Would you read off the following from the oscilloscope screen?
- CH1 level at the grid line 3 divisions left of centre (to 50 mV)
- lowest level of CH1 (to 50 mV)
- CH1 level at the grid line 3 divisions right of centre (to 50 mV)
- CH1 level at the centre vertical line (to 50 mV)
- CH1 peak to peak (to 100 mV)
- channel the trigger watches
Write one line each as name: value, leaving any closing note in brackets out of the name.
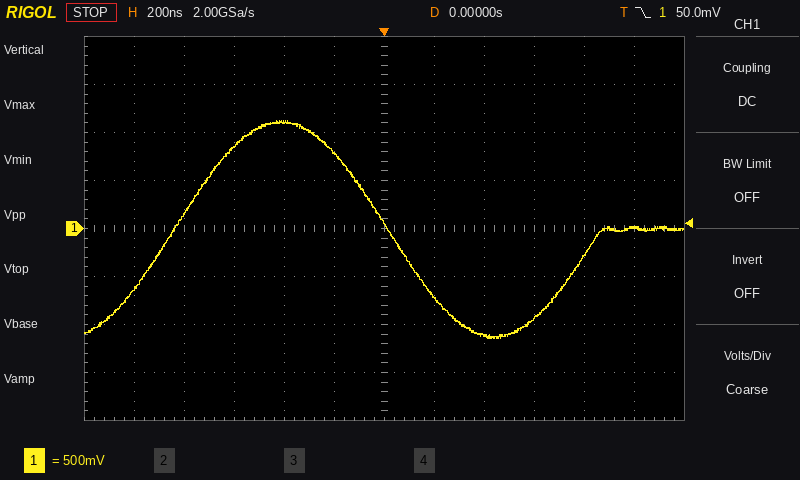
CH1 level at the grid line 3 divisions left of centre: 850 mV
lowest level of CH1: -1.15 V
CH1 level at the grid line 3 divisions right of centre: -950 mV
CH1 level at the centre vertical line: 50 mV
CH1 peak to peak: 2.30 V
channel the trigger watches: CH1
